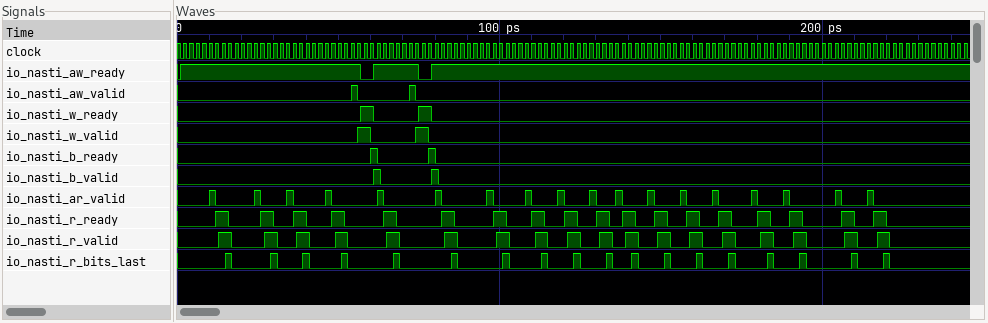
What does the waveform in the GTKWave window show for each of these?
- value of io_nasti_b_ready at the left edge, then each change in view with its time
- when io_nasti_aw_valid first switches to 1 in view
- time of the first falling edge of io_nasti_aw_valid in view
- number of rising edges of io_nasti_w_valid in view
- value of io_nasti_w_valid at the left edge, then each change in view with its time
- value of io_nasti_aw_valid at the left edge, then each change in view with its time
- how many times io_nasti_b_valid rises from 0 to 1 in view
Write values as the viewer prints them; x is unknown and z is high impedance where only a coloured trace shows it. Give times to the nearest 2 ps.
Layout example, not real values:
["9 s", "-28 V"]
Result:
["0, 1 at 60 ps, 0 at 62 ps, 1 at 78 ps, 0 at 80 ps", "54 ps", "56 ps", "2", "0, 1 at 56 ps, 0 at 60 ps, 1 at 74 ps, 0 at 78 ps", "0, 1 at 54 ps, 0 at 56 ps, 1 at 72 ps, 0 at 74 ps", "2"]
